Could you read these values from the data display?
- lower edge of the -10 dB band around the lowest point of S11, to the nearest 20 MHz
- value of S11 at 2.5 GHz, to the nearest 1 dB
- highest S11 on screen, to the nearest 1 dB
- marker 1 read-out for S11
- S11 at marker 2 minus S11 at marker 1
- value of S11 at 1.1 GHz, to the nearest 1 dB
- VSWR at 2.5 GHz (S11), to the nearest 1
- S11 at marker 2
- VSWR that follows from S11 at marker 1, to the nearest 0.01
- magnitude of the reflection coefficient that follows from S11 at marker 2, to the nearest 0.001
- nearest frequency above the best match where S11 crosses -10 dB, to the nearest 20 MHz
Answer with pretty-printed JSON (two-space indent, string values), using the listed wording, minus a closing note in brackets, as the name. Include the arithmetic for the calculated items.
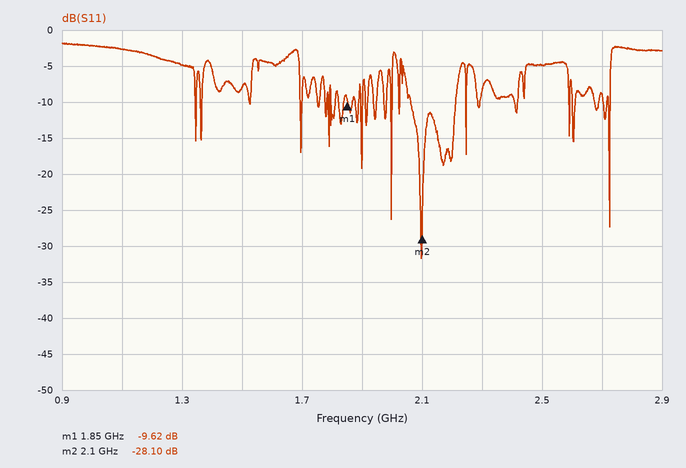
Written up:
{
  "lower edge of the -10 dB band around the lowest point of S11, to the nearest 20 MHz": "2.06 GHz",
  "value of S11 at 2.5 GHz, to the nearest 1 dB": "-5 dB",
  "highest S11 on screen, to the nearest 1 dB": "-2 dB",
  "marker 1 read-out for S11": "-9.62 dB",
  "S11 at marker 2 minus S11 at marker 1": "-28.1 − (-9.62) = -18.48 dB",
  "value of S11 at 1.1 GHz, to the nearest 1 dB": "-3 dB",
  "VSWR at 2.5 GHz (S11), to the nearest 1": "|Γ| = 10^(-5/20) = 0.5623; VSWR = (1 + 0.5623)/(1 − 0.5623) ≈ 4",
  "S11 at marker 2": "-28.10 dB",
  "VSWR that follows from S11 at marker 1, to the nearest 0.01": "(1 + 0.3304)/(1 − 0.3304) ≈ 1.99",
  "magnitude of the reflection coefficient that follows from S11 at marker 2, to the nearest 0.001": "10^(-28.1/20) ≈ 0.039",
  "nearest frequency above the best match where S11 crosses -10 dB, to the nearest 20 MHz": "2.22 GHz"
}
